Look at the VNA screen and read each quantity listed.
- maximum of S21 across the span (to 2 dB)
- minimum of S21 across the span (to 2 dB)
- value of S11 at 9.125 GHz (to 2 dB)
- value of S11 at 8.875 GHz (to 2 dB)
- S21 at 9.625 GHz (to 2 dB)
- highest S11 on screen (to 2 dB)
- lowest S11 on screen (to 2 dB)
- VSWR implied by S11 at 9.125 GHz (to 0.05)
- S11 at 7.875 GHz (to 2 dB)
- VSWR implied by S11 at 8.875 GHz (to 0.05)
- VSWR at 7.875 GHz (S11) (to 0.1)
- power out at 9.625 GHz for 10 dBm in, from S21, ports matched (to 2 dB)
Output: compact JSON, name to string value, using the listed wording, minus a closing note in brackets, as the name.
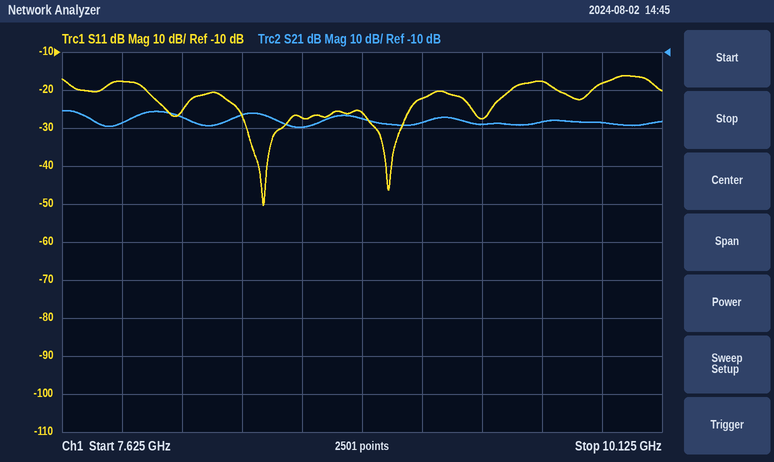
{"maximum of S21 across the span": "-26 dB", "minimum of S21 across the span": "-30 dB", "value of S11 at 9.125 GHz": "-22 dB", "value of S11 at 8.875 GHz": "-26 dB", "S21 at 9.625 GHz": "-28 dB", "highest S11 on screen": "-16 dB", "lowest S11 on screen": "-50 dB", "VSWR implied by S11 at 9.125 GHz": "1.15", "S11 at 7.875 GHz": "-18 dB", "VSWR implied by S11 at 8.875 GHz": "1.10", "VSWR at 7.875 GHz (S11)": "1.3", "power out at 9.625 GHz for 10 dBm in, from S21, ports matched": "-18 dBm"}
